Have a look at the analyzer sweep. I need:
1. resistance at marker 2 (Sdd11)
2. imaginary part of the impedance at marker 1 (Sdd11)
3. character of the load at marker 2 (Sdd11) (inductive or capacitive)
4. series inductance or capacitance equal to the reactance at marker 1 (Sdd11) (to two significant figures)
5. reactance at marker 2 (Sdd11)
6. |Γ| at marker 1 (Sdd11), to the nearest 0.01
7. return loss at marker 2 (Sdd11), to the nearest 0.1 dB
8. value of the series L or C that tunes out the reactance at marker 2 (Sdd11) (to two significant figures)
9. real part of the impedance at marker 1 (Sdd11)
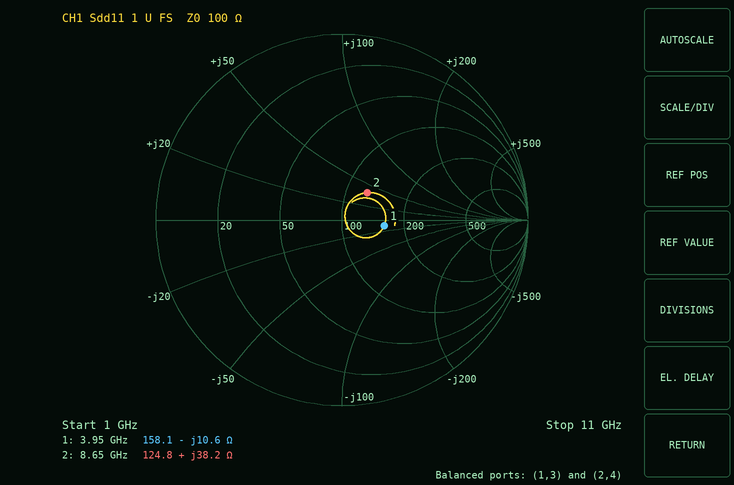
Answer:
124.8 Ω
-10.6 Ω
inductive
3.8 pF
+38.2 Ω
0.23
14.0 dB
480 fF
158.1 Ω
